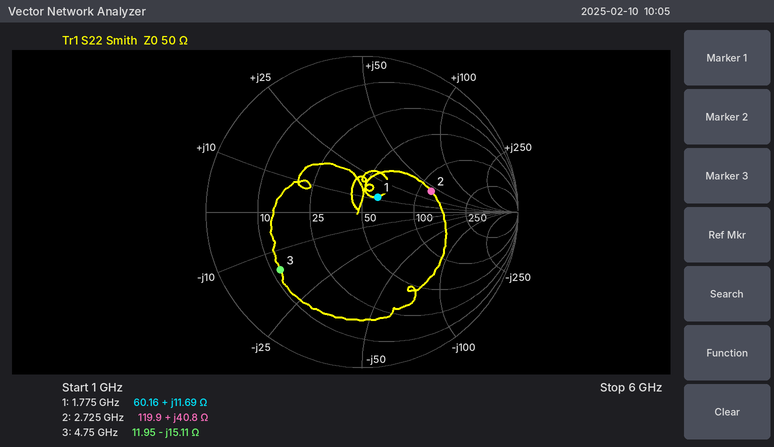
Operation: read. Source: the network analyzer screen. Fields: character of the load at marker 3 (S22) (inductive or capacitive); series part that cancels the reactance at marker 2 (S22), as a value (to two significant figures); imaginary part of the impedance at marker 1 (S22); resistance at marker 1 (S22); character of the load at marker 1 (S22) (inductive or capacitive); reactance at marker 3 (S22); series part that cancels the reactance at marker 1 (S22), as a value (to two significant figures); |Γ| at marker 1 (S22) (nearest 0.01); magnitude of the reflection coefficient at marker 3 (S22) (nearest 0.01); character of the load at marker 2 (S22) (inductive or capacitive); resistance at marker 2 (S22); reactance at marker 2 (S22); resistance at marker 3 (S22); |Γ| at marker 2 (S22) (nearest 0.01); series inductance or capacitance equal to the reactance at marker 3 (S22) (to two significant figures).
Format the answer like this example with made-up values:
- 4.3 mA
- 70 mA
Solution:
- capacitive
- 1.4 pF
- +11.69 Ω
- 60.16 Ω
- inductive
- -15.11 Ω
- 7.7 pF
- 0.14
- 0.64
- inductive
- 119.9 Ω
- +40.8 Ω
- 11.95 Ω
- 0.46
- 2.2 pF
